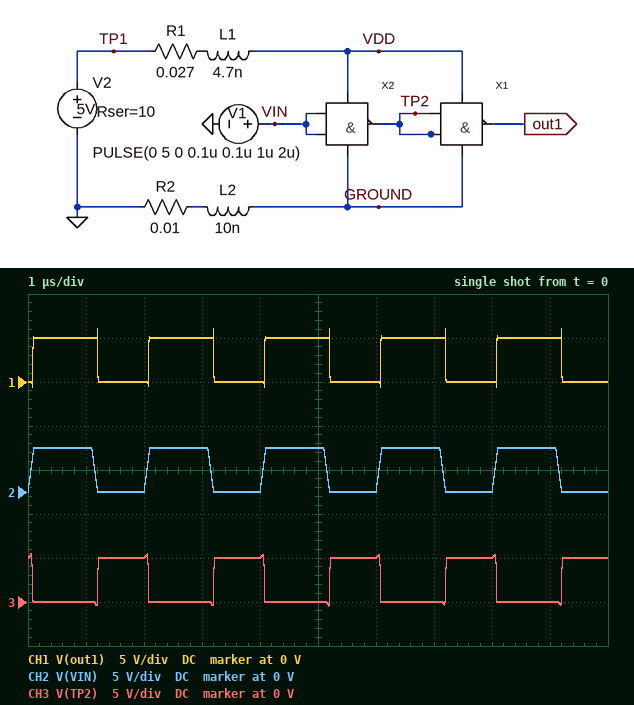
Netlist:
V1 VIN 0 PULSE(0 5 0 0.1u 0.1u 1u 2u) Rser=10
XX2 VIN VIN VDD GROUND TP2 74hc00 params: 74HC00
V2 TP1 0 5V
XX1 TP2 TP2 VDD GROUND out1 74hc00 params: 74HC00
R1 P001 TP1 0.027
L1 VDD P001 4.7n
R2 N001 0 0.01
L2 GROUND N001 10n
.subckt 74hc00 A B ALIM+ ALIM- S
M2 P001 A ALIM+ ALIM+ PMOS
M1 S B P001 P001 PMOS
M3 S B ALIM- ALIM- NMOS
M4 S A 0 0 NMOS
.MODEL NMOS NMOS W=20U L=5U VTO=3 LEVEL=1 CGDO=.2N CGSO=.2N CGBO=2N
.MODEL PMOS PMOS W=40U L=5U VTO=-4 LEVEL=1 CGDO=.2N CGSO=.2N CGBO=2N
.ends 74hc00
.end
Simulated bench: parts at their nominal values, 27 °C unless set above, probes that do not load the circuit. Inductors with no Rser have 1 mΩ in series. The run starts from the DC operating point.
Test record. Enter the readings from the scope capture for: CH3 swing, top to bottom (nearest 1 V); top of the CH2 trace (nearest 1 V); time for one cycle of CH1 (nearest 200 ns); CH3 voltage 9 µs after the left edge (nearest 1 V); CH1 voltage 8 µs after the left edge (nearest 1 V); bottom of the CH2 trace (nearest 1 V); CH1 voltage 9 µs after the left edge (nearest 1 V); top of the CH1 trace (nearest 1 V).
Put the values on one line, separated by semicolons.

6 V; 5 V; 2.0 µs; 0 V; 0 V; 0 V; 5 V; 6 V
